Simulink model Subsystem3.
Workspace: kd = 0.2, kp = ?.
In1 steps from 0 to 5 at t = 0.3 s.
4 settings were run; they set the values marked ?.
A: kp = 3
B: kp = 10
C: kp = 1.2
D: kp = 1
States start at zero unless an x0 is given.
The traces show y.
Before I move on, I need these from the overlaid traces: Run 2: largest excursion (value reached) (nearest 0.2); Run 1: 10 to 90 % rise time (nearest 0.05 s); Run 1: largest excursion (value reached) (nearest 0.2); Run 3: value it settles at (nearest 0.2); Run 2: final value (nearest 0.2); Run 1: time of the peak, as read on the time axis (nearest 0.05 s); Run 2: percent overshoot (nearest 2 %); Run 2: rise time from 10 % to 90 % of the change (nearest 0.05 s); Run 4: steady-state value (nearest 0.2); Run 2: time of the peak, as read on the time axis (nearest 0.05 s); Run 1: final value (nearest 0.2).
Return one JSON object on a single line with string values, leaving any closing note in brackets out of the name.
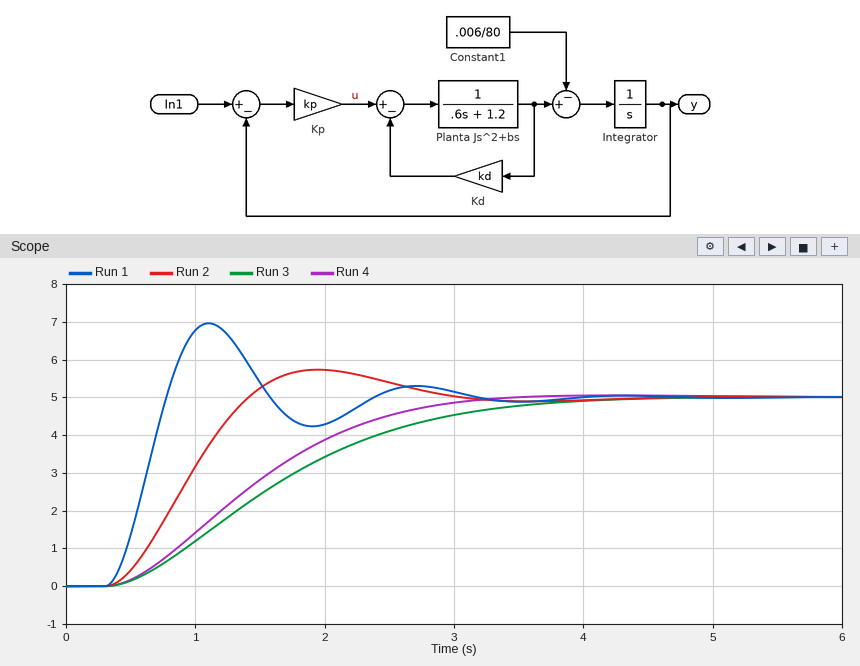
{"Run 2: largest excursion (value reached)": "5.8", "Run 1: 10 to 90 % rise time": "0.30 s", "Run 1: largest excursion (value reached)": "7.0", "Run 3: value it settles at": "5.0", "Run 2: final value": "5.0", "Run 1: time of the peak, as read on the time axis": "1.10 s", "Run 2: percent overshoot": "14 %", "Run 2: rise time from 10 % to 90 % of the change": "0.75 s", "Run 4: steady-state value": "5.0", "Run 2: time of the peak, as read on the time axis": "1.95 s", "Run 1: final value": "5.0"}
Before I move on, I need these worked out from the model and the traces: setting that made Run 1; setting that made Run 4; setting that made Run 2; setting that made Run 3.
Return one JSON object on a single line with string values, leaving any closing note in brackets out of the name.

{"setting that made Run 1": "B", "setting that made Run 4": "C", "setting that made Run 2": "A", "setting that made Run 3": "D"}
